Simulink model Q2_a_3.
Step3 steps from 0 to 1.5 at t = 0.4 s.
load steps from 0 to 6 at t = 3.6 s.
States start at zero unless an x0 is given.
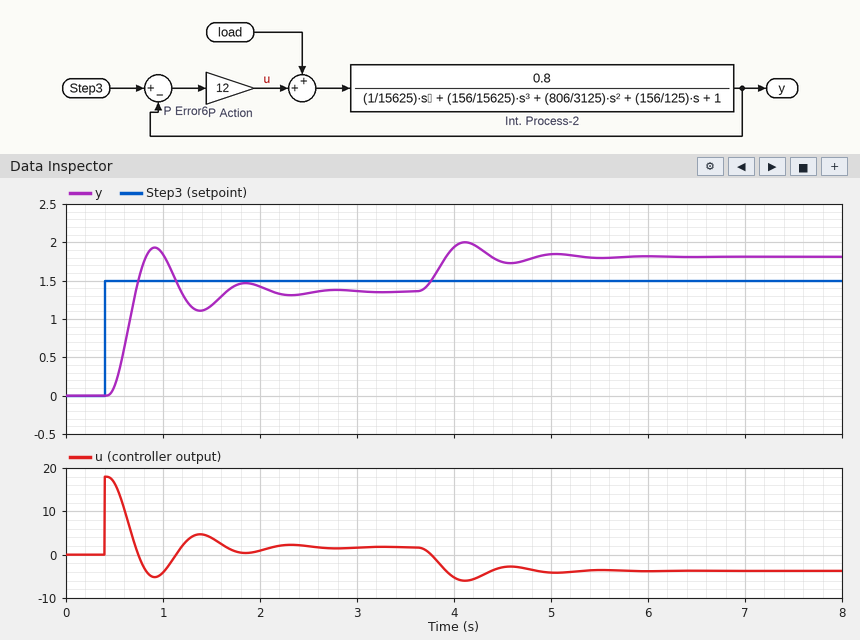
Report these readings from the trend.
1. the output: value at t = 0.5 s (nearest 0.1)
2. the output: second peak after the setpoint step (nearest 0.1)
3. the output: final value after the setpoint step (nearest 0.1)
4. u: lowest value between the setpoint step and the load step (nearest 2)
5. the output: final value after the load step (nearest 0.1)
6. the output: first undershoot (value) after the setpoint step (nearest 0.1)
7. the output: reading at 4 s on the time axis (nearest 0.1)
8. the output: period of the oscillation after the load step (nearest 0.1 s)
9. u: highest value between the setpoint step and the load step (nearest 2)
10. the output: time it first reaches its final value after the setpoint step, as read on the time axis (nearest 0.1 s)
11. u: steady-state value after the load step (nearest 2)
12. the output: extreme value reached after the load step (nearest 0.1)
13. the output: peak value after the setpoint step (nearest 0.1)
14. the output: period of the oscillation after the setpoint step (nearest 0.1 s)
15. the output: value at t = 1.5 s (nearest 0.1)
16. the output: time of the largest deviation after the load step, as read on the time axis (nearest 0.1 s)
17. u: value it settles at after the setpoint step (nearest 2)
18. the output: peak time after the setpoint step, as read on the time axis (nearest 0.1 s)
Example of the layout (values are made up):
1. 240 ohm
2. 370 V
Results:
1. 0.1
2. 1.5
3. 1.4
4. -6
5. 1.8
6. 1.1
7. 1.9
8. 0.9 s
9. 18
10. 0.7 s
11. -4
12. 2.0
13. 1.9
14. 0.9 s
15. 1.2
16. 4.1 s
17. 2
18. 0.9 s
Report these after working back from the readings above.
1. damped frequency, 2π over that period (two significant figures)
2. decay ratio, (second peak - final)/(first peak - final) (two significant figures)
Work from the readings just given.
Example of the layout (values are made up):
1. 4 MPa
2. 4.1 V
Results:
1. 7.0 rad/s
2. 0.20
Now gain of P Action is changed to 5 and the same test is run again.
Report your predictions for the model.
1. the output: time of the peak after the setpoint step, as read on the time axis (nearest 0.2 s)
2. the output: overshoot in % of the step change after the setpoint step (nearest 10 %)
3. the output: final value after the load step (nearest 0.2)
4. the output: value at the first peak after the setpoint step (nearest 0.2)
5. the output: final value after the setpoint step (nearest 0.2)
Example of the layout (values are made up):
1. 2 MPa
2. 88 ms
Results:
1. 1.2 s
2. 20 %
3. 2.2
4. 1.4
5. 1.2
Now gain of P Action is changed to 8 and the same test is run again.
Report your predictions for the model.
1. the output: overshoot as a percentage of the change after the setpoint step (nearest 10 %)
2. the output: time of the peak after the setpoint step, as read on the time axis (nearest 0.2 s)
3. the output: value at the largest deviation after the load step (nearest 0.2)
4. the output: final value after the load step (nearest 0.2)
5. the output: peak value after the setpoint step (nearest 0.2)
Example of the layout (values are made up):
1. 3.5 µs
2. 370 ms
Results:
1. 30 %
2. 1.0 s
3. 2.2
4. 2.0
5. 1.6
